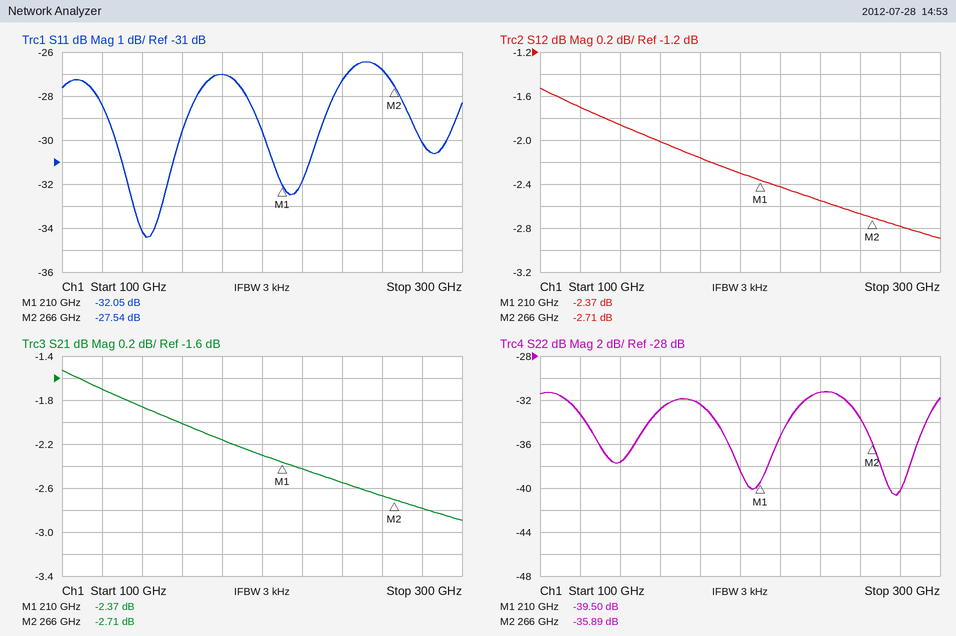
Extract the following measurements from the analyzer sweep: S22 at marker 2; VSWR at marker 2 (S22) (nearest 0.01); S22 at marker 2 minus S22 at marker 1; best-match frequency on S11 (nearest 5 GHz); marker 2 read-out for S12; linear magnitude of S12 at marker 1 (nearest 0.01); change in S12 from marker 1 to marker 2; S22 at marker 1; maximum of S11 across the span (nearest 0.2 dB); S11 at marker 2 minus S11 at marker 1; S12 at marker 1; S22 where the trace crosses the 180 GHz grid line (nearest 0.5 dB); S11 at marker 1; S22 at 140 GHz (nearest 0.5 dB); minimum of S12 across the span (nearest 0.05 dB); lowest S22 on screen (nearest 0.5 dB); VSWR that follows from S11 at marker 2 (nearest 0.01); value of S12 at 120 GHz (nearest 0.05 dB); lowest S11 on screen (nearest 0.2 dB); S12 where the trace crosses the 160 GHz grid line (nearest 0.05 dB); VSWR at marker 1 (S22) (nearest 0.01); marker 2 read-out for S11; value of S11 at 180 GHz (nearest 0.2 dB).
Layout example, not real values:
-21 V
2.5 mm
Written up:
-35.89 dB
1.03
3.61 dB
140 GHz
-2.71 dB
0.76
-0.34 dB
-39.50 dB
-26.4 dB
4.51 dB
-2.37 dB
-32.5 dB
-32.05 dB
-37.5 dB
-2.90 dB
-40.5 dB
1.09
-1.70 dB
-34.4 dB
-2.00 dB
1.02
-27.54 dB
-27.0 dB
